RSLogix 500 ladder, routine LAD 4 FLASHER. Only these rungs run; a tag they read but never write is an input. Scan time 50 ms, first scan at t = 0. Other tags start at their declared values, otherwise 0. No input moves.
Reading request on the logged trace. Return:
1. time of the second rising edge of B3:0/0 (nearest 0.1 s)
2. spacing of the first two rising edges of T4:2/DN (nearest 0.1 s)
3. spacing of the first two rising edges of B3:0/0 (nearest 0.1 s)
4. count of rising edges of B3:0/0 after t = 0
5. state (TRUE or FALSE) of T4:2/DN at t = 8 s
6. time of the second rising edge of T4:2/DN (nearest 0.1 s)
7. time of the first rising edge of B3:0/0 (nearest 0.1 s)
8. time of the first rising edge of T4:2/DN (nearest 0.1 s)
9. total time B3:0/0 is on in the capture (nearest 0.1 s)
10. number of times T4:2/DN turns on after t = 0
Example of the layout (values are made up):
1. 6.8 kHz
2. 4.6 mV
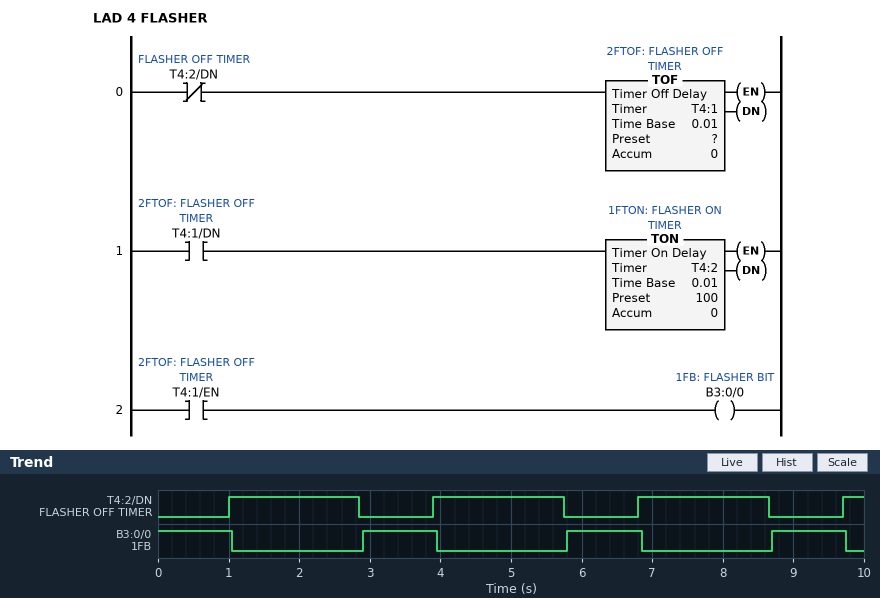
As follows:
1. 5.8 s
2. 2.9 s
3. 2.9 s
4. 3
5. TRUE
6. 3.9 s
7. 2.9 s
8. 1.0 s
9. 4.2 s
10. 4
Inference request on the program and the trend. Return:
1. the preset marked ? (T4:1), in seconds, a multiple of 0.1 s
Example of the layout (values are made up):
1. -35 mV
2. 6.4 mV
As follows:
1. 1.8 s
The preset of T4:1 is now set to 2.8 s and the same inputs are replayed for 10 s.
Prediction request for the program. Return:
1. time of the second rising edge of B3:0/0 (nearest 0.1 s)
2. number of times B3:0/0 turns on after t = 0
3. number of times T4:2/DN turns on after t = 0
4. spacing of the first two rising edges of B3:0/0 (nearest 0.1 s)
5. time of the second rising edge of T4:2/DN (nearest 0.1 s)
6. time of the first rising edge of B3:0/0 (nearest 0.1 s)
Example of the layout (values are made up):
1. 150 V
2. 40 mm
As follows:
1. 7.8 s
2. 2
3. 3
4. 3.9 s
5. 4.9 s
6. 3.9 s
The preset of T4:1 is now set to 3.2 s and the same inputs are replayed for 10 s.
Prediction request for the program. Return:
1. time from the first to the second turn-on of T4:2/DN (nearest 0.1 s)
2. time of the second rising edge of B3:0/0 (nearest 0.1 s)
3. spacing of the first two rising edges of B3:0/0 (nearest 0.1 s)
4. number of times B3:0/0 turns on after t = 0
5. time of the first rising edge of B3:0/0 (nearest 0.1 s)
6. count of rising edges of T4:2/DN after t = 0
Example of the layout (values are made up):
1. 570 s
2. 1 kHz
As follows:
1. 4.3 s
2. 8.6 s
3. 4.3 s
4. 2
5. 4.3 s
6. 3
